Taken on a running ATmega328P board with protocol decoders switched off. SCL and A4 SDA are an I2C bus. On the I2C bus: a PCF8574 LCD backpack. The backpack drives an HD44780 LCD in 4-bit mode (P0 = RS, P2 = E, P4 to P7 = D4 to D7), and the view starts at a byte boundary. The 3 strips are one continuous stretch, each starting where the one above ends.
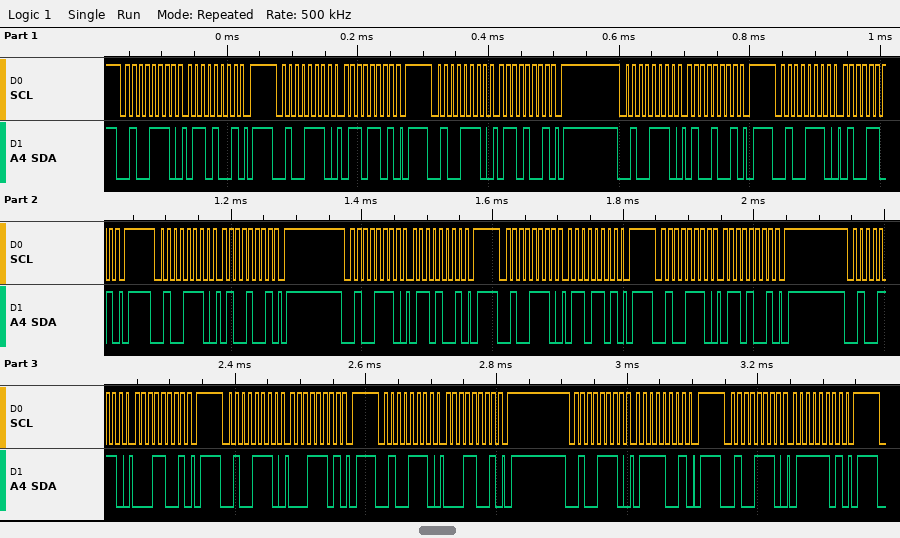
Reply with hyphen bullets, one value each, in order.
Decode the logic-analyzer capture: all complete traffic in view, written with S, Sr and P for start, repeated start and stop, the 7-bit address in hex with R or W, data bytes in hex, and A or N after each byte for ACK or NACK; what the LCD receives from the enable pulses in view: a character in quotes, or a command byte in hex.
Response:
- S 27W A 69 A P S 27W A 6D A P S 27W A 69 A P S 27W A 49 A P S 27W A 4D A P S 27W A 49 A P S 27W A 69 A P S 27W A 6D A P S 27W A 69 A P S 27W A 19 A P S 27W A 1D A P S 27W A 19 A P S 27W A 79 A P S 27W A 7D A P
- 'd' 'a'
